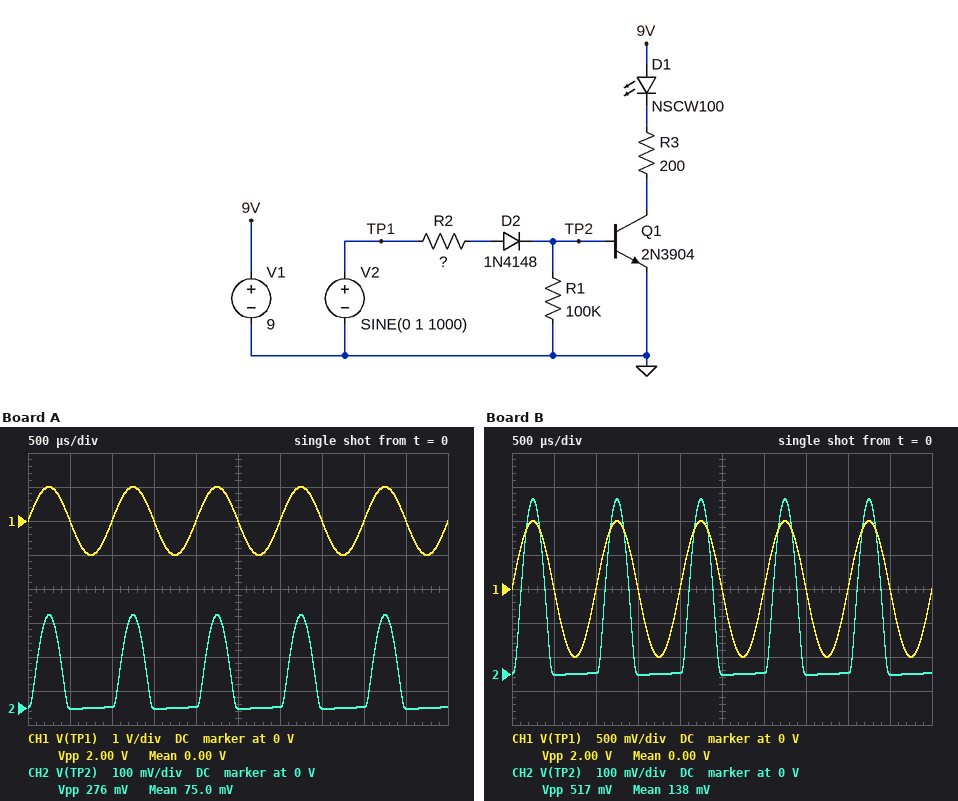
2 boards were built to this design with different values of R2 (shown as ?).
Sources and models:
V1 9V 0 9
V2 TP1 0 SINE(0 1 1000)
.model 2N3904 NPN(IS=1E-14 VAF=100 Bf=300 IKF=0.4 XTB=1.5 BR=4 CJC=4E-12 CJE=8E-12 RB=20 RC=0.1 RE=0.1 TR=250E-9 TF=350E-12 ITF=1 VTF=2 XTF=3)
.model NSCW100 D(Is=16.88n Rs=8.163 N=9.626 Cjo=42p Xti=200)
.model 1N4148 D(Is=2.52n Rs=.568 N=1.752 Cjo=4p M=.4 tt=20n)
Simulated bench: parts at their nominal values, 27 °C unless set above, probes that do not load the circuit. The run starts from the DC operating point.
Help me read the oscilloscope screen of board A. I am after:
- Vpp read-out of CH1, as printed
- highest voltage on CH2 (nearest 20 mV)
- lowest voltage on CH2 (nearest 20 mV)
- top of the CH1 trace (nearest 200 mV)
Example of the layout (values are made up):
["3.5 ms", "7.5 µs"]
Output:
["2.00 V", "280 mV", "0 V", "1.0 V"]
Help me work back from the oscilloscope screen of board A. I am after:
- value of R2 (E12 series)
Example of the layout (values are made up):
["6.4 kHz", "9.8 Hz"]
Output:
["150 kΩ"]
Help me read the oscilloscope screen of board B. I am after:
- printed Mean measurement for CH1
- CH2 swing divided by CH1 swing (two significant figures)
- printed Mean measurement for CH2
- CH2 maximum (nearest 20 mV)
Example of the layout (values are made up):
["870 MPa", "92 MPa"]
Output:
["0.00 V", "0.26", "138 mV", "520 mV"]
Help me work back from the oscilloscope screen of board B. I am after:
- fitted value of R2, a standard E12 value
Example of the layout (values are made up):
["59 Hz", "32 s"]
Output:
["27 kΩ"]
